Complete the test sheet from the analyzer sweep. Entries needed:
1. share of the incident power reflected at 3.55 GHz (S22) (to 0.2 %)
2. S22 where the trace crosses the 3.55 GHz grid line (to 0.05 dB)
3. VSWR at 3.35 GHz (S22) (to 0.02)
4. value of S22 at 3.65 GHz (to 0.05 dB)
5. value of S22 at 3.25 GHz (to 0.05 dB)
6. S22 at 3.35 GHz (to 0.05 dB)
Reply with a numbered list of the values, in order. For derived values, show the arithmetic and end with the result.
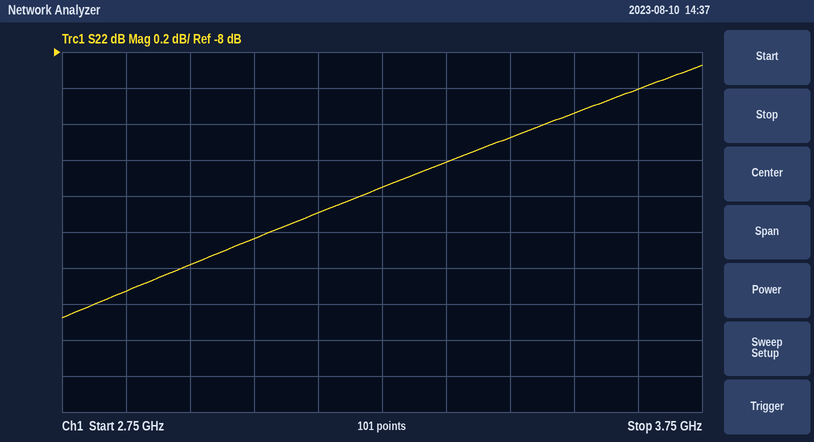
1. 10^(-8.35/10) ≈ 14.6 %
2. -8.35 dB
3. |Γ| = 10^(-8.6/20) = 0.3715; VSWR = (1 + 0.3715)/(1 − 0.3715) ≈ 2.18
4. -8.20 dB
5. -8.75 dB
6. -8.60 dB
